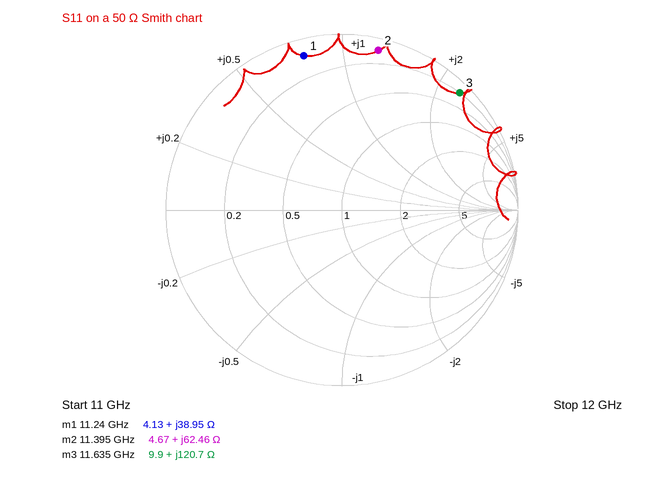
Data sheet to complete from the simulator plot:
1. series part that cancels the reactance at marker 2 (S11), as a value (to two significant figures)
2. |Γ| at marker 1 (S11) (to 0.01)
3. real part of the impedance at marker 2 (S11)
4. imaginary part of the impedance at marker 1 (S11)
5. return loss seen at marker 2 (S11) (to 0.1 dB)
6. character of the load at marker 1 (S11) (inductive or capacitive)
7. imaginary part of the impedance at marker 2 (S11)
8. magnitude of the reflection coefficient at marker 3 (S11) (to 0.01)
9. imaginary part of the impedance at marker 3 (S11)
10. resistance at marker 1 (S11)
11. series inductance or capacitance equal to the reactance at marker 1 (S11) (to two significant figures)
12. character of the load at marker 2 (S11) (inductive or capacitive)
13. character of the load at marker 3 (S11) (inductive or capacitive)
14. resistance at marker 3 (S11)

220 fF
0.90
4.67 Ω
+38.95 Ω
0.6 dB
inductive
+62.46 Ω
0.94
+120.7 Ω
4.13 Ω
550 pH
inductive
inductive
9.9 Ω
